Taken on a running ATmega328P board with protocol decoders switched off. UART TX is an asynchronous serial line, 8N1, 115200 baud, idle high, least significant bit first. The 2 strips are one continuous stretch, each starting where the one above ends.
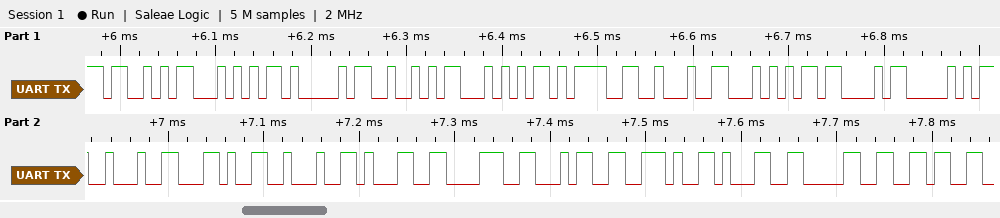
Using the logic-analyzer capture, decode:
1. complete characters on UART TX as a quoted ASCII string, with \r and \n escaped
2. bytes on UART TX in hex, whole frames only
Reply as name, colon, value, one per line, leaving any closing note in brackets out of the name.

complete characters on UART TX as a quoted ASCII string, with \r and \n escaped: "START=\"TCP\",\"184.106"
bytes on UART TX in hex, whole frames only: 53 54 41 52 54 3D 22 54 43 50 22 2C 22 31 38 34 2E 31 30 36
